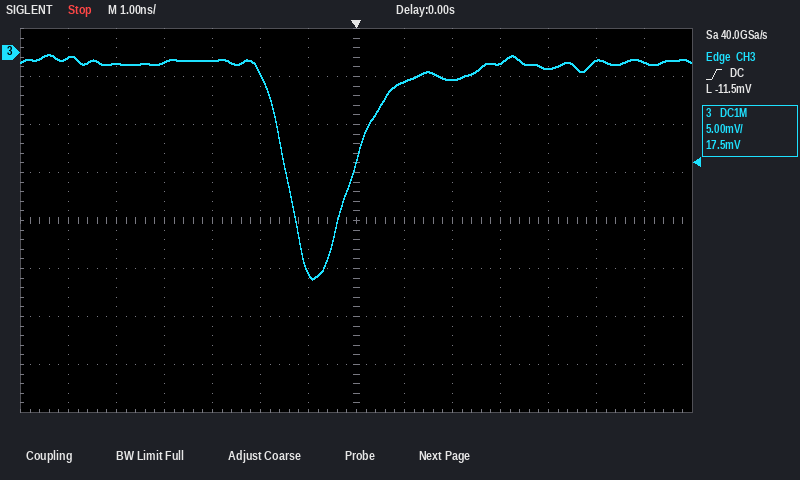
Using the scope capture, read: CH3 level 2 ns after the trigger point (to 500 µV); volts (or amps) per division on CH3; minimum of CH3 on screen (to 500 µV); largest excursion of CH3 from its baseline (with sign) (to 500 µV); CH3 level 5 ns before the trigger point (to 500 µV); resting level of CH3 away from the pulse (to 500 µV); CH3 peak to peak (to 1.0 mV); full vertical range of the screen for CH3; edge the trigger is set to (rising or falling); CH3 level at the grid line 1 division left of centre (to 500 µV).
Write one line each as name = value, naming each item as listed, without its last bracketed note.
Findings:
CH3 level 2 ns after the trigger point = -3.0 mV
volts (or amps) per division on CH3 = 5 mV
minimum of CH3 on screen = -23.5 mV
largest excursion of CH3 from its baseline (with sign) = -22.5 mV
CH3 level 5 ns before the trigger point = -1.0 mV
resting level of CH3 away from the pulse = -1.0 mV
CH3 peak to peak = 23.0 mV
full vertical range of the screen for CH3 = 40 mV
edge the trigger is set to = rising
CH3 level at the grid line 1 division left of centre = -23.0 mV
